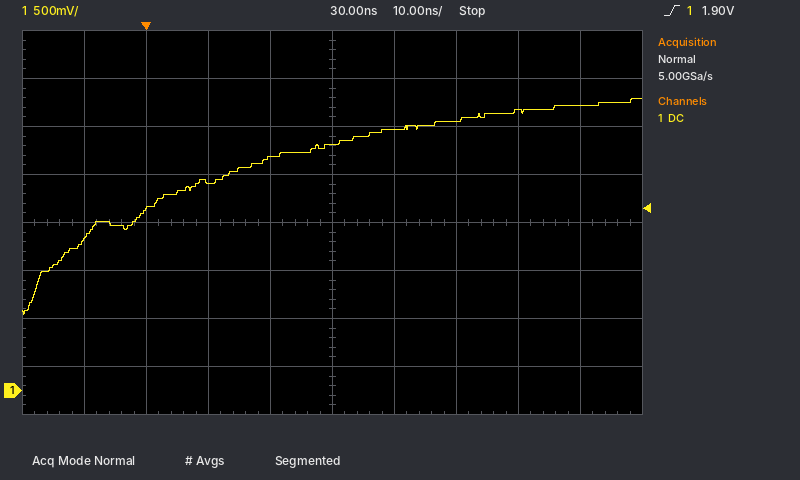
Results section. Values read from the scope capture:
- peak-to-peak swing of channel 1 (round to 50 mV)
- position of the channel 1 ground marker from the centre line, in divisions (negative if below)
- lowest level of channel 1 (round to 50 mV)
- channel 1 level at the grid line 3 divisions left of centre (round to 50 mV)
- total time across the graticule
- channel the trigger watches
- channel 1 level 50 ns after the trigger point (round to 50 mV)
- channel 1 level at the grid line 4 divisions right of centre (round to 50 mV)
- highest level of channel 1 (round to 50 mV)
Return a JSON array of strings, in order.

["2.25 V", "-3.5 div", "800 mV", "1.90 V", "100 ns", "channel 1", "2.80 V", "2.95 V", "3.05 V"]
